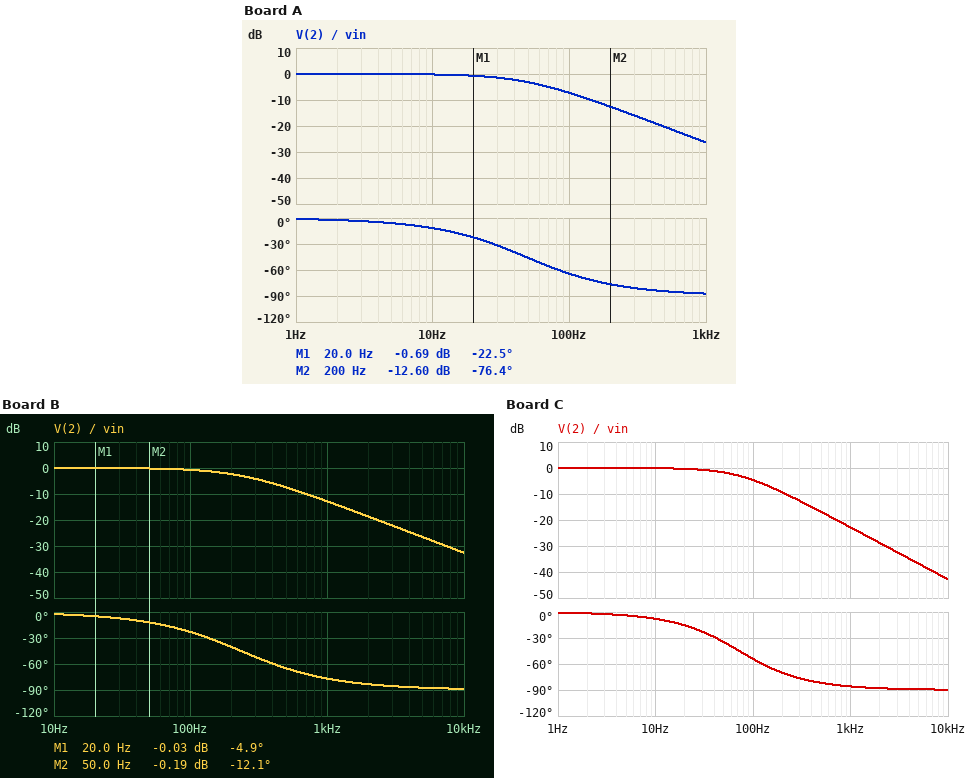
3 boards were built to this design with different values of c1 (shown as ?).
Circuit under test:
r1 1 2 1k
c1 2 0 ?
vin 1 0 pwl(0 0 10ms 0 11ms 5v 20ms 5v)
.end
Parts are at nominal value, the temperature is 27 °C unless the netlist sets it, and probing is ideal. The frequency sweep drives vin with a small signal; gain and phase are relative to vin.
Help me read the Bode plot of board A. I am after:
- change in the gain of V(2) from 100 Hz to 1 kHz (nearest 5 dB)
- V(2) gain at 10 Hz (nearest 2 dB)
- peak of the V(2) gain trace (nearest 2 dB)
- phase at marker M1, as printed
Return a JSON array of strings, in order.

["-20 dB", "0 dB", "0 dB", "-22.5 deg"]
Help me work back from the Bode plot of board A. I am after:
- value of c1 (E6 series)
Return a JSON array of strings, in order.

["3.3 µF"]
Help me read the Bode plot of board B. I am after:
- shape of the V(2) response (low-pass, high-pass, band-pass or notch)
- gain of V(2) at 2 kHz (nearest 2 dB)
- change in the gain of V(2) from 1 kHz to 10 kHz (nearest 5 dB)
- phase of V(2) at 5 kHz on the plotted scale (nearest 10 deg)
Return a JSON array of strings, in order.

["low-pass", "-18 dB", "-20 dB", "-90 deg"]
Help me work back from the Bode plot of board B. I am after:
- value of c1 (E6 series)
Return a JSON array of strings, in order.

["680 nF"]
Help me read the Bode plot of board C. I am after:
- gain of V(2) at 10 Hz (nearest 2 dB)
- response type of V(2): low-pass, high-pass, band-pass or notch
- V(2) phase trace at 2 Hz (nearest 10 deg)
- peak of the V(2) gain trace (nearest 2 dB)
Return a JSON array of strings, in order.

["0 dB", "low-pass", "0 deg", "0 dB"]
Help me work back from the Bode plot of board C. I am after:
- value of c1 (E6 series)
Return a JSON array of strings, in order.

["2.2 µF"]
